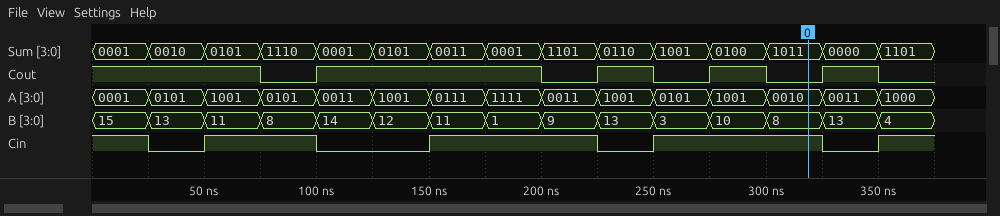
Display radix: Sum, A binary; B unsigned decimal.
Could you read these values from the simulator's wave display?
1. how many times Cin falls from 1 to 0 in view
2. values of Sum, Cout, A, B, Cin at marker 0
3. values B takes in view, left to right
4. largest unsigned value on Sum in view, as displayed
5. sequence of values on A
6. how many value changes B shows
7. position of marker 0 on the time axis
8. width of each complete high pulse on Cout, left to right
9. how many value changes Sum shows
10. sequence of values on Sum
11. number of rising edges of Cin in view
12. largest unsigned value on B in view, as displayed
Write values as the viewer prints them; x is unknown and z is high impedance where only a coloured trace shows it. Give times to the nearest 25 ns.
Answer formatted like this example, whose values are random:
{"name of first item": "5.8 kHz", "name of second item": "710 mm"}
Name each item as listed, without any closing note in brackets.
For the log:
{"how many times Cin falls from 1 to 0 in view": "4", "values of Sum, Cout, A, B, Cin at marker 0": "Sum=1011, Cout=0, A=0010, B=8, Cin=1", "values B takes in view, left to right": "15, 13, 11, 8, 14, 12, 11, 1, 9, 13, 3, 10, 8, 13, 4", "largest unsigned value on Sum in view, as displayed": "1110", "sequence of values on A": "0001, 0101, 1001, 0101, 0011, 1001, 0111, 1111, 0011, 1001, 0101, 1001, 0010, 0011, 1000", "how many value changes B shows": "14", "position of marker 0 on the time axis": "325 ns", "width of each complete high pulse on Cout, left to right": "100 ns, 25 ns, 25 ns, 25 ns", "how many value changes Sum shows": "14", "sequence of values on Sum": "0001, 0010, 0101, 1110, 0001, 0101, 0011, 0001, 1101, 0110, 1001, 0100, 1011, 0000, 1101", "number of rising edges of Cin in view": "4", "largest unsigned value on B in view, as displayed": "15"}
